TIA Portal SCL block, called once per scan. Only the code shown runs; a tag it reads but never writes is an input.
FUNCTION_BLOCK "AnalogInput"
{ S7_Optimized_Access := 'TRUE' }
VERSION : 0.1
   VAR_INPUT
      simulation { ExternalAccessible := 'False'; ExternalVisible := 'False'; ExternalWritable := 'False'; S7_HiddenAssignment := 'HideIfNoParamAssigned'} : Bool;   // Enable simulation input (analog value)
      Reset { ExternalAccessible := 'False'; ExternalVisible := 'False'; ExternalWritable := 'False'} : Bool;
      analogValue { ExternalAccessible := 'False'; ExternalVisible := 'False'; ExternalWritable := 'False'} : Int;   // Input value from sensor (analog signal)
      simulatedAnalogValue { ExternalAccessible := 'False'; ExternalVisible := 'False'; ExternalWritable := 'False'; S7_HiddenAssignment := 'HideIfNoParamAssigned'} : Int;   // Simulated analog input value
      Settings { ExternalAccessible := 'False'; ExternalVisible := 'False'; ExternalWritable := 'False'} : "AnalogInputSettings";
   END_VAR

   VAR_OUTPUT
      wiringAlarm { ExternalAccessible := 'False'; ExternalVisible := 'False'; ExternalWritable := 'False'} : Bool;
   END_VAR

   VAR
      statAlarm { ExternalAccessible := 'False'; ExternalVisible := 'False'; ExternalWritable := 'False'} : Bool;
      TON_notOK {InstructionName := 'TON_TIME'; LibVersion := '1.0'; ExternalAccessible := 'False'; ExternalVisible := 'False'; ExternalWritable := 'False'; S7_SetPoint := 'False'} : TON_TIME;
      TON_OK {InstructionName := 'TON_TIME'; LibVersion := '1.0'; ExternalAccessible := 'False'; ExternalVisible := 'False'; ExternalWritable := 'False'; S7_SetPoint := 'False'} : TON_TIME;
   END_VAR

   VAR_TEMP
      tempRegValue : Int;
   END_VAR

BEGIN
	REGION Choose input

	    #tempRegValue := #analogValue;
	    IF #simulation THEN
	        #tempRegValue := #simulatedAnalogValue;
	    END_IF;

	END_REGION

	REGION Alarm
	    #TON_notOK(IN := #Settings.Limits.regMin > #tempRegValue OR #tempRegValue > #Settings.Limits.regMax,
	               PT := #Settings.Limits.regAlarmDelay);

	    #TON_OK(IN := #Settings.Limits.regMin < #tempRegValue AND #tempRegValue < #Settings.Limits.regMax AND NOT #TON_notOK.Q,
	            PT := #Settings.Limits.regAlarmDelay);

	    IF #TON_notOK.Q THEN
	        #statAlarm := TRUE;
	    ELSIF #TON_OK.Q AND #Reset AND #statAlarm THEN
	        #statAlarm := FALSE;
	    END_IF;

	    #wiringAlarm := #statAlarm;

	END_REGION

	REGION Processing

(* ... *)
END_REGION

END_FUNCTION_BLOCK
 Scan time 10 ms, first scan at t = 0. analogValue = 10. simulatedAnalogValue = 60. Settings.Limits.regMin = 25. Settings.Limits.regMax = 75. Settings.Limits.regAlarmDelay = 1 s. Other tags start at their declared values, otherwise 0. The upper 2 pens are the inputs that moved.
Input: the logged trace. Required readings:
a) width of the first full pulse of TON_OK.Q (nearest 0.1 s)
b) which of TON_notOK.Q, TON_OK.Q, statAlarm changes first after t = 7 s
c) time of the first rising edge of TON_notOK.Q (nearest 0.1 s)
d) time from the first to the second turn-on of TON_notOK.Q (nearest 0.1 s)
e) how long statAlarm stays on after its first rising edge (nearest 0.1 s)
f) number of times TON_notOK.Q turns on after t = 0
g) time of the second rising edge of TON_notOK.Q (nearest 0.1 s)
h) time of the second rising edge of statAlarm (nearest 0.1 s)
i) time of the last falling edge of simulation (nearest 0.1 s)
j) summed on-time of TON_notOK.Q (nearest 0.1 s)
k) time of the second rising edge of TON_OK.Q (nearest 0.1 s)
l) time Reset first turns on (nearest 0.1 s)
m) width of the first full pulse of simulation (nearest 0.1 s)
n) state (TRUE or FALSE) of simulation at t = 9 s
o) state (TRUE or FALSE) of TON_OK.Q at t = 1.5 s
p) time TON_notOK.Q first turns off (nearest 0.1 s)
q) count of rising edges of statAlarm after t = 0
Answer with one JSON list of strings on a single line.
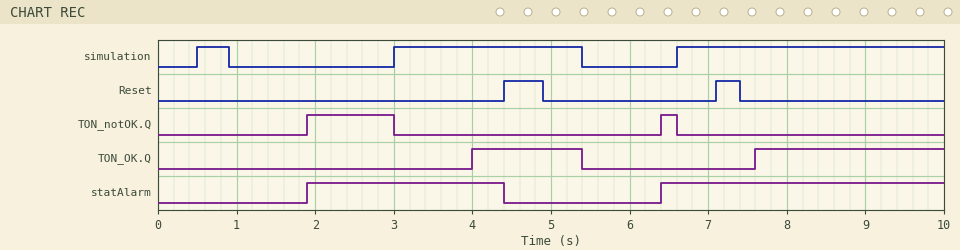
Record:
["1.4 s", "TON_OK.Q", "1.9 s", "4.5 s", "2.5 s", "2", "6.4 s", "6.4 s", "5.4 s", "1.3 s", "7.6 s", "4.4 s", "0.4 s", "TRUE", "FALSE", "3.0 s", "2"]
